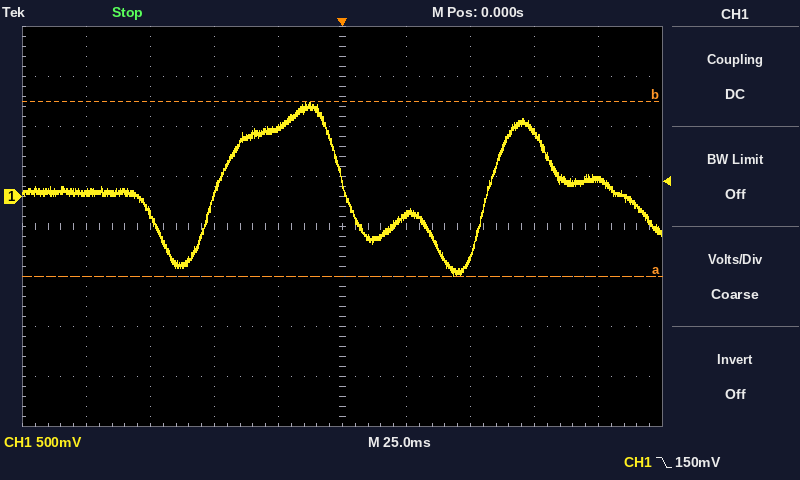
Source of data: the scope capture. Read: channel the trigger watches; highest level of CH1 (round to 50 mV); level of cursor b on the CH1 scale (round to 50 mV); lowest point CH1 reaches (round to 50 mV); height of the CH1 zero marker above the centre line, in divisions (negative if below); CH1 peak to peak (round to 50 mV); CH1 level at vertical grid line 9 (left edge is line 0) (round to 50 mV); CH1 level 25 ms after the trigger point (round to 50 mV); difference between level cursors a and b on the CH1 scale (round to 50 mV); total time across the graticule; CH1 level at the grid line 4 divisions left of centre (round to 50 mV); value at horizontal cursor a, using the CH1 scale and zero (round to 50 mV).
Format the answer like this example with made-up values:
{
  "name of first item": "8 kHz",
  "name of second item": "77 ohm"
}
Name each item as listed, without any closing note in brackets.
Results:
{
  "channel the trigger watches": "CH1",
  "highest level of CH1": "950 mV",
  "level of cursor b on the CH1 scale": "950 mV",
  "lowest point CH1 reaches": "-800 mV",
  "height of the CH1 zero marker above the centre line, in divisions": "+0.6 div",
  "CH1 peak to peak": "1.75 V",
  "CH1 level at vertical grid line 9 (left edge is line 0)": "150 mV",
  "CH1 level 25 ms after the trigger point": "-200 mV",
  "difference between level cursors a and b on the CH1 scale": "1.75 V",
  "total time across the graticule": "250 ms",
  "CH1 level at the grid line 4 divisions left of centre": "50 mV",
  "value at horizontal cursor a, using the CH1 scale and zero": "-800 mV"
}
